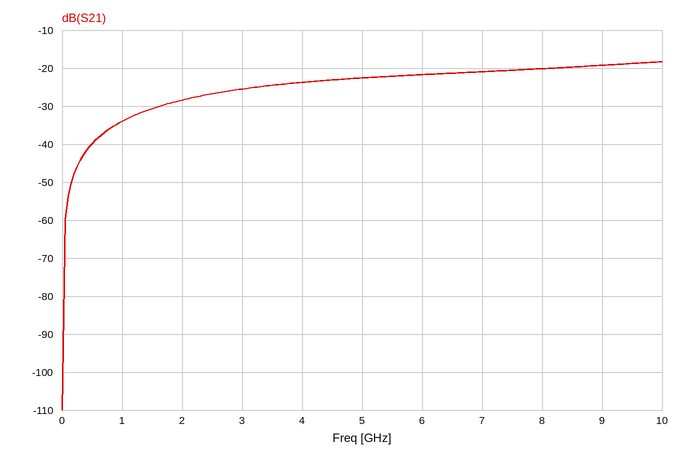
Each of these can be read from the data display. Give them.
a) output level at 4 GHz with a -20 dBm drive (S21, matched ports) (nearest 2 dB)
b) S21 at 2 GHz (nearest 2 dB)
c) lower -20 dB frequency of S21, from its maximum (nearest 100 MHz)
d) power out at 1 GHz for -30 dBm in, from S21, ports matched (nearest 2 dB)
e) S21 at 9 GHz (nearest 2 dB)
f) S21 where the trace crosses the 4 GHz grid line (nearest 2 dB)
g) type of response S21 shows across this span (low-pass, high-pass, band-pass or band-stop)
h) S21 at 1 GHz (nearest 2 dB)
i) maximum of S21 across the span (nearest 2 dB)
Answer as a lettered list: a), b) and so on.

a) -44 dBm
b) -28 dB
c) 600 MHz
d) -64 dBm
e) -20 dB
f) -24 dB
g) high-pass
h) -34 dB
i) -18 dB
